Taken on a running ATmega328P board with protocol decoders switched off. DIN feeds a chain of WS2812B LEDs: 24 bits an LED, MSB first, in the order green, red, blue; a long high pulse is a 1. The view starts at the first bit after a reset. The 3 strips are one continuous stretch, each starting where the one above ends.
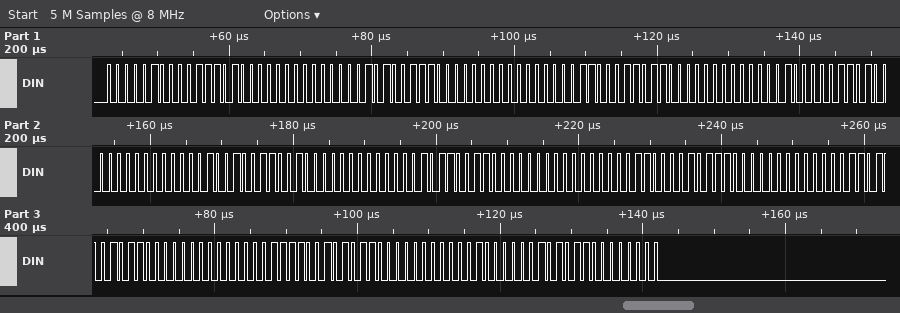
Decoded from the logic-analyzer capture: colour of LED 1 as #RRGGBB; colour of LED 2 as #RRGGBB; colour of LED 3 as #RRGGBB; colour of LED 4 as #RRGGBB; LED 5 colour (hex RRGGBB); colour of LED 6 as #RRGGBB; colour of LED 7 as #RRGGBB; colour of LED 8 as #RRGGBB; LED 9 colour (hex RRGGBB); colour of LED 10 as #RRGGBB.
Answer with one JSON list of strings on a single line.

["#3A0400", "#380500", "#360600", "#340800", "#320900", "#300B00", "#2E0C00", "#2C0D00", "#2B0F00", "#2B1000"]
